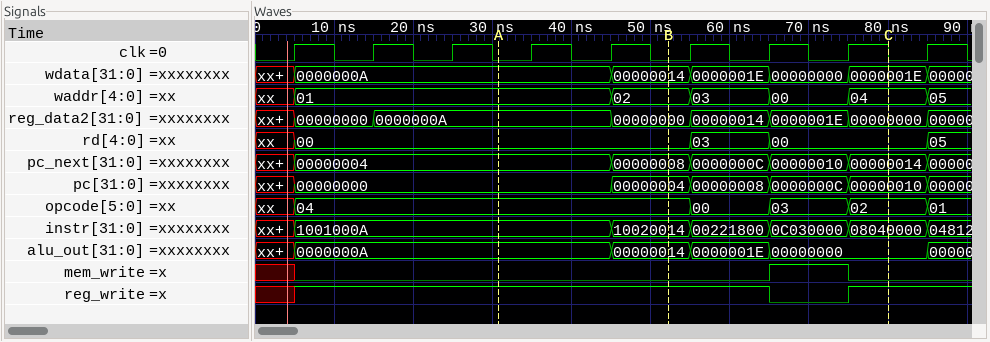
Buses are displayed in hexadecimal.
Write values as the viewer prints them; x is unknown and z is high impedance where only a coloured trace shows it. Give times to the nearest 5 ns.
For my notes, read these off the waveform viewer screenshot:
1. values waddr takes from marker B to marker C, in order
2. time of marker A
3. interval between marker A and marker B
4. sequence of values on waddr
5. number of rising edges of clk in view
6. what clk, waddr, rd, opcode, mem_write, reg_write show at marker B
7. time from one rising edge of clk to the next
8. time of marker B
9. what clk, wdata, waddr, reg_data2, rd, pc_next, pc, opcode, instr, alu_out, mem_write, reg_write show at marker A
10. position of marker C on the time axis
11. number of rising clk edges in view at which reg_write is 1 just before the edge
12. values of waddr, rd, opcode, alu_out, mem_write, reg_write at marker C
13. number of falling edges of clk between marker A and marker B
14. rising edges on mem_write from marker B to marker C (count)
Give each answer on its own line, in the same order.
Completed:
02, 03, 00, 04
30 ns
20 ns
xx, 01, 02, 03, 00, 04, 05
9
clk=0, waddr=02, rd=00, opcode=04, mem_write=0, reg_write=1
10 ns
50 ns
clk=0, wdata=0000000A, waddr=01, reg_data2=0000000A, rd=00, pc_next=00000004, pc=00000000, opcode=04, instr=1001000A, alu_out=0000000A, mem_write=0, reg_write=1
80 ns
7
waddr=04, rd=00, opcode=02, alu_out=00000000, mem_write=0, reg_write=1
2
1
